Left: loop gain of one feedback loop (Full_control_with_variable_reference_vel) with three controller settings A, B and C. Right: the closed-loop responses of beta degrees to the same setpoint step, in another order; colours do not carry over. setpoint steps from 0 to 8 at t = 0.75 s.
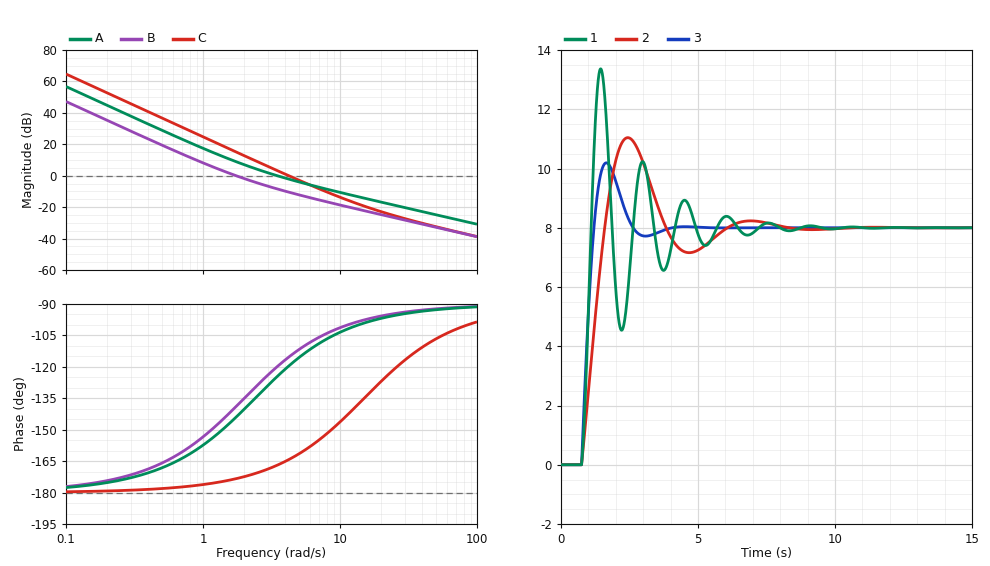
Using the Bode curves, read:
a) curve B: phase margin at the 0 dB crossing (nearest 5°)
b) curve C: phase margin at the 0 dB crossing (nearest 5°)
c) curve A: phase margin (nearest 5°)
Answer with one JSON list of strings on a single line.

["40°", "15°", "55°"]
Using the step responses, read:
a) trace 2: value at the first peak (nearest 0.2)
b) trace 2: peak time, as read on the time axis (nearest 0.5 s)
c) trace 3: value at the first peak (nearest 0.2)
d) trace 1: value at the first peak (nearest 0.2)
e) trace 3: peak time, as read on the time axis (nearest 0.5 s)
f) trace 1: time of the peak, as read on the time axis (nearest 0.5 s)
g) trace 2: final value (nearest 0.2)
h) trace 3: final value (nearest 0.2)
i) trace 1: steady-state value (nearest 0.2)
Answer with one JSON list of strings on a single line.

["11.0", "2.5 s", "10.2", "13.4", "1.5 s", "1.5 s", "8.0", "8.0", "8.0"]
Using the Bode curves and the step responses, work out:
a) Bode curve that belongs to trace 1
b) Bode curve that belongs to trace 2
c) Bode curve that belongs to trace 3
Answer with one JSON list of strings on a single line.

["C", "B", "A"]
